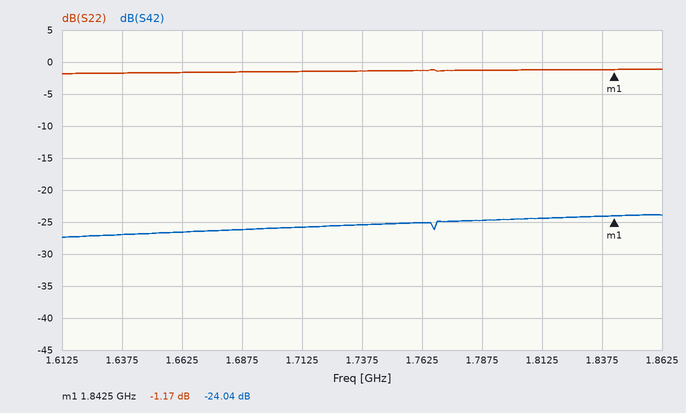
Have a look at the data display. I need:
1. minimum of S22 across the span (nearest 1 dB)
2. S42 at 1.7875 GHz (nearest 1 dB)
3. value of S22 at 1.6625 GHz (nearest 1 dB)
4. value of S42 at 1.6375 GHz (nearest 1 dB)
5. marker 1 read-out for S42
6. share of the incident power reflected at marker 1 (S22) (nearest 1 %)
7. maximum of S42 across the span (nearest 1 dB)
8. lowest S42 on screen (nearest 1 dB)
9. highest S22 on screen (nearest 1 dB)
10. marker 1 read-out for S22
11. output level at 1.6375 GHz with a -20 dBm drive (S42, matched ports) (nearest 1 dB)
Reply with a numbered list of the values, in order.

1. -2 dB
2. -25 dB
3. -2 dB
4. -27 dB
5. -24.04 dB
6. 76 %
7. -24 dB
8. -27 dB
9. -1 dB
10. -1.17 dB
11. -47 dBm
